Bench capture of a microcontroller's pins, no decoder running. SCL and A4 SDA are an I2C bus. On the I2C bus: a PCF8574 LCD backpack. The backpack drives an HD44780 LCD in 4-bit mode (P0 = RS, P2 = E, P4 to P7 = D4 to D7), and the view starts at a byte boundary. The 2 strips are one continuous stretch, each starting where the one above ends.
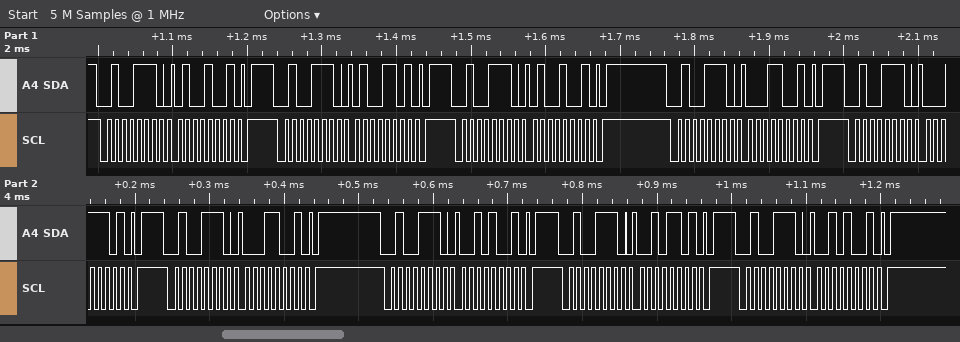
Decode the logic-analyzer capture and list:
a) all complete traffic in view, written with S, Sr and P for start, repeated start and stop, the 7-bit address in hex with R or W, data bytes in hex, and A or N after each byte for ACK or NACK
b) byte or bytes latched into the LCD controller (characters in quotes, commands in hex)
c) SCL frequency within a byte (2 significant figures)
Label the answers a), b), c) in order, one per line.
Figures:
a) S 27W A 49 A P S 27W A 4D A P S 27W A 49 A P S 27W A 19 A P S 27W A 1D A P S 27W A 19 A P S 27W A 29 A P S 27W A 2D A P S 27W A 29 A P
b) 'A'
c) 100 kHz
